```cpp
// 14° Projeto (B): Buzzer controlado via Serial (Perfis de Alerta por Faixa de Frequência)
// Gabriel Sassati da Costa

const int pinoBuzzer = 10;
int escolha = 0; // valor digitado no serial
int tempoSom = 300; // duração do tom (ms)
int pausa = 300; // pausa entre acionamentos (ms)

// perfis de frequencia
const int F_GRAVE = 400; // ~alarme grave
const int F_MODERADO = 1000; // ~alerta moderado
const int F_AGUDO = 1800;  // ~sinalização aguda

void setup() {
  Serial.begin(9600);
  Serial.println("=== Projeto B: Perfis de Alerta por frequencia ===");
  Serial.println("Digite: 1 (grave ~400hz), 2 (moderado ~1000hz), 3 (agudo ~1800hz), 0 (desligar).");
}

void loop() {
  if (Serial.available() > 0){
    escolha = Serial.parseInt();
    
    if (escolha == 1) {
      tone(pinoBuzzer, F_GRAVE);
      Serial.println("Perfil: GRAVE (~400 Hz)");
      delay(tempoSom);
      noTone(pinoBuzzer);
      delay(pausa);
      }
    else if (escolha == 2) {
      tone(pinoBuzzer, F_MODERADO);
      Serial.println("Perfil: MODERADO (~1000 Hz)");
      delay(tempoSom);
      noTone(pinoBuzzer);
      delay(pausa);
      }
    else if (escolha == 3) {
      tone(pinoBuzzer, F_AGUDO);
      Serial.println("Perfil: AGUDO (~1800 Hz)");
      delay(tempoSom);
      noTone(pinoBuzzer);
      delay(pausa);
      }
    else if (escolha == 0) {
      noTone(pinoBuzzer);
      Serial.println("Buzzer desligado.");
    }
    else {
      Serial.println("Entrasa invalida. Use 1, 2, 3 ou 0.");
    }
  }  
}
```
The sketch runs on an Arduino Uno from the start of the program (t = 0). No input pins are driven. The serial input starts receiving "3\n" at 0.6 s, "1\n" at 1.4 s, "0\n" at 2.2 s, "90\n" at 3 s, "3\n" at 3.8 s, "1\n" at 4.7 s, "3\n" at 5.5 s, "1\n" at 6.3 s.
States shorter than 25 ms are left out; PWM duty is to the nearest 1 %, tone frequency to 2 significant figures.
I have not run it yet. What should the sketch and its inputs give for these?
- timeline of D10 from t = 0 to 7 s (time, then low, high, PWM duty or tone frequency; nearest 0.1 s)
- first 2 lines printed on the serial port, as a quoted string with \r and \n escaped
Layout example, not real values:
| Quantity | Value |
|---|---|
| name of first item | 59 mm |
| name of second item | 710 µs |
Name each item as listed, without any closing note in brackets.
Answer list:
| Quantity | Value |
|---|---|
| timeline of D10 from t = 0 to 7 s | 0.6 s tone 1800 Hz; 0.9 s low; 1.4 s tone 400 Hz; 1.7 s low; 3.8 s tone 1800 Hz; 4.1 s low; 4.7 s tone 400 Hz; 5 s low; 5.5 s tone 1800 Hz; 5.8 s low; 6.3 s tone 400 Hz; 6.6 s low |
| first 2 lines printed on the serial port, as a quoted string with \r and \n escaped | "=== Projeto B: Perfis de Alerta por frequencia ===\r\nDigite: 1 (grave ~400hz), 2 (moderado ~1000hz), 3 (agudo ~1800hz), 0 (desligar).\r\n" |
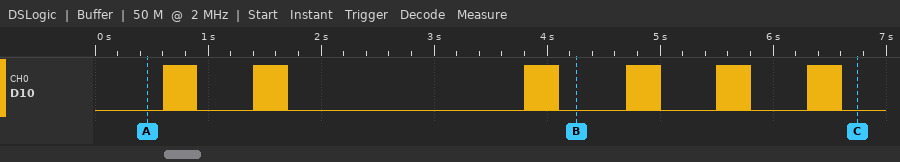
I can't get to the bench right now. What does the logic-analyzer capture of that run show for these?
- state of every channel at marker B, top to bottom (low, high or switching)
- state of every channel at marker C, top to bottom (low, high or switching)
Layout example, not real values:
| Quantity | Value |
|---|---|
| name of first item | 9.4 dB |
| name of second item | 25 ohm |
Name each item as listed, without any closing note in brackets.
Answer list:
| Quantity | Value |
|---|---|
| state of every channel at marker B, top to bottom | D10 low |
| state of every channel at marker C, top to bottom | D10 low |
